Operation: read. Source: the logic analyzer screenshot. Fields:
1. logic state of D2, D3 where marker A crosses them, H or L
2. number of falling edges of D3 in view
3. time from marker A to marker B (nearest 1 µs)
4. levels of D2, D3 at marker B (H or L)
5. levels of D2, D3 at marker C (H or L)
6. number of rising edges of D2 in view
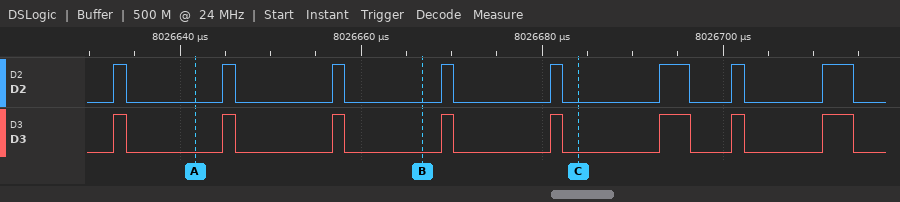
D2=L, D3=L
8
25 µs
D2=L, D3=L
D2=L, D3=L
8
